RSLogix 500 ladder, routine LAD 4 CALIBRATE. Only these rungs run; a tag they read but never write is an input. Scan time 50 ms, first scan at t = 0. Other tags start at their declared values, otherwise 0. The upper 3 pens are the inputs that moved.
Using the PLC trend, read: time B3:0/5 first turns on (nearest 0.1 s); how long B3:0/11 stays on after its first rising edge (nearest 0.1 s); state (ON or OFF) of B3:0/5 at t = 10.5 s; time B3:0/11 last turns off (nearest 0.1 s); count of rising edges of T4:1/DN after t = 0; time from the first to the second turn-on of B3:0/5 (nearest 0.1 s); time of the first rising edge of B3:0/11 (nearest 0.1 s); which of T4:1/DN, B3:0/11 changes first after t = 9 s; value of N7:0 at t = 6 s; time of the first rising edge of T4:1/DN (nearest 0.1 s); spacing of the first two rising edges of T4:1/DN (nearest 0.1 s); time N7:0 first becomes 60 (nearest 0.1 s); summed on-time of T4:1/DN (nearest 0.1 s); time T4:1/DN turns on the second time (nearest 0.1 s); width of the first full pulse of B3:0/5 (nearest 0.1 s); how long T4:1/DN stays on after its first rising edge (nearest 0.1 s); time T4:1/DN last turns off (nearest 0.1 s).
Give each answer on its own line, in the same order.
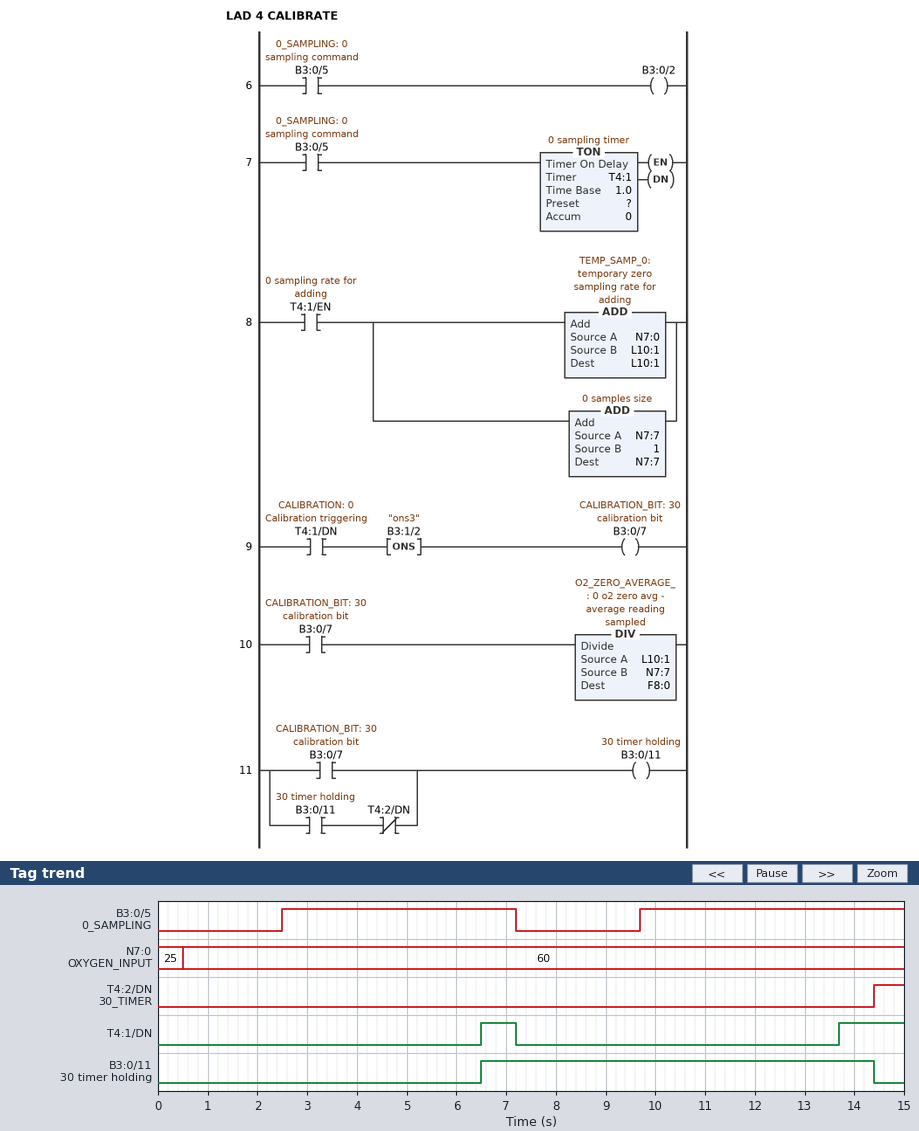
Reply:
2.5 s
7.9 s
ON
14.4 s
2
7.2 s
6.5 s
T4:1/DN
60
6.5 s
7.2 s
0.5 s
2.0 s
13.7 s
4.7 s
0.7 s
7.2 s
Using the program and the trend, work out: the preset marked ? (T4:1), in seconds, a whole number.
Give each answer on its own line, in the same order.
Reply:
4 s
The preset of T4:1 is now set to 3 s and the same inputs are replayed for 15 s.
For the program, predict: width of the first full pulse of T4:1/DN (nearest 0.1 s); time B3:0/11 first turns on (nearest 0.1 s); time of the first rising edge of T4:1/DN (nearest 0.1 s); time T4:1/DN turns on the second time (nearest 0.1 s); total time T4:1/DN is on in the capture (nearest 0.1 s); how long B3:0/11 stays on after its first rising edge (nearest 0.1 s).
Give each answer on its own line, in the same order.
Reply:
1.7 s
5.5 s
5.5 s
12.7 s
4.0 s
8.9 s
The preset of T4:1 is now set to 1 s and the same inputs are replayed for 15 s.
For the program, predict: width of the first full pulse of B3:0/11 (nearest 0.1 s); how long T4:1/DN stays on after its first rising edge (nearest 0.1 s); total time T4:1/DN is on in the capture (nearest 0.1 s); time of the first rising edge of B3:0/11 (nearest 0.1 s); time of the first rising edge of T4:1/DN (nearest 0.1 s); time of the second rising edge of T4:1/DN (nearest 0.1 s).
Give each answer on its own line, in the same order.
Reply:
10.9 s
3.7 s
8.0 s
3.5 s
3.5 s
10.7 s
